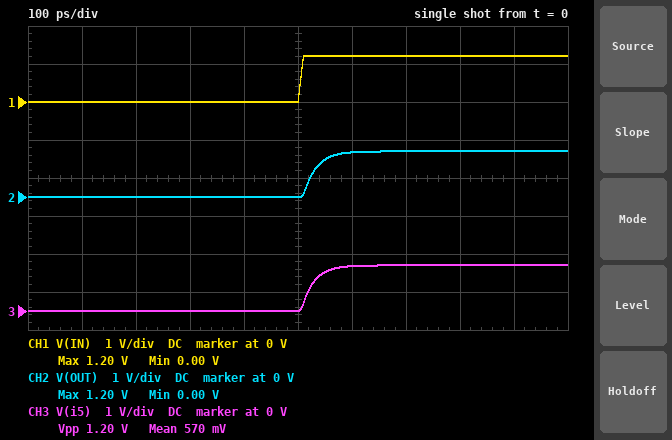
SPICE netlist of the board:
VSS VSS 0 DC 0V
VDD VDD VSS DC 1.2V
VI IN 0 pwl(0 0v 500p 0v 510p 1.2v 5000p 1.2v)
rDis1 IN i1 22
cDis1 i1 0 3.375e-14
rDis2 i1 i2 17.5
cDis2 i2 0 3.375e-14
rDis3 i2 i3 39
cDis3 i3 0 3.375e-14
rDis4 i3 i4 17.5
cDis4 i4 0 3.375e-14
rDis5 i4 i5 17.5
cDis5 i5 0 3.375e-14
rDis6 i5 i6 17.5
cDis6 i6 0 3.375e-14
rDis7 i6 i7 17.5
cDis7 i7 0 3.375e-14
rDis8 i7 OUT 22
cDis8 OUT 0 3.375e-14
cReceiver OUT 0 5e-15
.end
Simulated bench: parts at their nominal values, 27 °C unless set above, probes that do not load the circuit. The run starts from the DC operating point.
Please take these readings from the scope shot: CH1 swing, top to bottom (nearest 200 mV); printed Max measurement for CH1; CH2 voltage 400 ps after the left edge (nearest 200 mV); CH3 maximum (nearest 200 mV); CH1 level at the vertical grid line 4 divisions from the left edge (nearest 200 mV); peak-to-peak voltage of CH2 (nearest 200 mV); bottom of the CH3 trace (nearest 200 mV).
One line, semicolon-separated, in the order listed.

1.2 V; 1.20 V; 0 V; 1.2 V; 0 V; 1.2 V; 0 V
